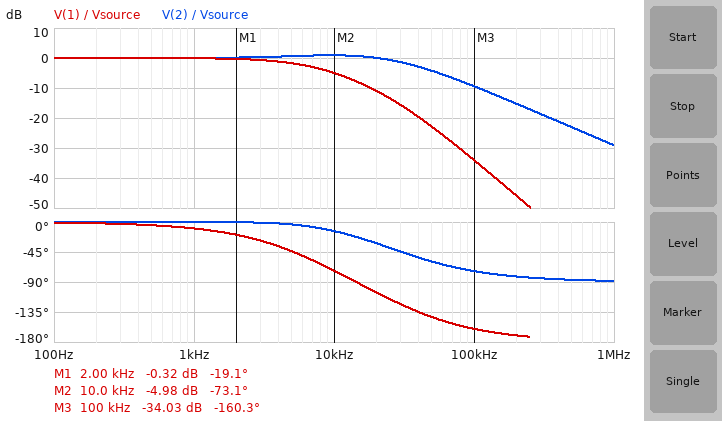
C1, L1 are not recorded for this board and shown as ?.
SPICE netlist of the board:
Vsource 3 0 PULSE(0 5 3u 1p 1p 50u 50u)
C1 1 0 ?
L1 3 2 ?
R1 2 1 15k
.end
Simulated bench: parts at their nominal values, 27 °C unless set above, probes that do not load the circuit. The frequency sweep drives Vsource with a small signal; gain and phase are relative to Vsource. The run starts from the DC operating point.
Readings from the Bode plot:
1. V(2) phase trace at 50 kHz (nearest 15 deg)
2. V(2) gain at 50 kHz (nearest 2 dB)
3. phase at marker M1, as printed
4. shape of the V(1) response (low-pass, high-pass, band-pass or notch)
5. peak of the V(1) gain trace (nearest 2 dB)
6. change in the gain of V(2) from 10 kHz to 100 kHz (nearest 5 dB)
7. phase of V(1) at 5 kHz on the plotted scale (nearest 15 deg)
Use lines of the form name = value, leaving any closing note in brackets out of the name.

V(2) phase trace at 50 kHz = -60 deg
V(2) gain at 50 kHz = -4 dB
phase at marker M1, as printed = -19.1 deg
shape of the V(1) response = low-pass
peak of the V(1) gain trace = 0 dB
change in the gain of V(2) from 10 kHz to 100 kHz = -10 dB
phase of V(1) at 5 kHz on the plotted scale = -45 deg
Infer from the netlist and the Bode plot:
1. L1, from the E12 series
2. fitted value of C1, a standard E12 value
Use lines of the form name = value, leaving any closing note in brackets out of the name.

L1, from the E12 series = 68 mH
fitted value of C1, a standard E12 value = 1.8 nF
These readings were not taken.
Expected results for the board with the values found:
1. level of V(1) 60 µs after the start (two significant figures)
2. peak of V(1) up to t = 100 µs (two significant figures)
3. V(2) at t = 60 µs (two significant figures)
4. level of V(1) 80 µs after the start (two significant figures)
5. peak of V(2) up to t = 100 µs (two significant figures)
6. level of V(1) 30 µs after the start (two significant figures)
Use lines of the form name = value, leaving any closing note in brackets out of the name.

level of V(1) 60 µs after the start = 4.5 V
peak of V(1) up to t = 100 µs = 4.9 V
V(2) at t = 60 µs = 5.1 V
level of V(1) 80 µs after the start = 4.8 V
peak of V(2) up to t = 100 µs = 5.5 V
level of V(1) 30 µs after the start = 3.1 V
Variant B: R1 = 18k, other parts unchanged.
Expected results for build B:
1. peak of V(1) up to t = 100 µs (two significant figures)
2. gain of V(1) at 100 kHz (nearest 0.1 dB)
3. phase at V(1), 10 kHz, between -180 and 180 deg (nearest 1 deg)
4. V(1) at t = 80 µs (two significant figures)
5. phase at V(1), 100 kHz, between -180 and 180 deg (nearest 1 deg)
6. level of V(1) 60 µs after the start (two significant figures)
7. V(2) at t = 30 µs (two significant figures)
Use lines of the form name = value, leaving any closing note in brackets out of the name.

peak of V(1) up to t = 100 µs = 4.8 V
gain of V(1) at 100 kHz = -34.2 dB
phase at V(1), 10 kHz, between -180 and 180 deg = -76 deg
V(1) at t = 80 µs = 4.6 V
phase at V(1), 100 kHz, between -180 and 180 deg = -157 deg
level of V(1) 60 µs after the start = 4.2 V
V(2) at t = 30 µs = 5.3 V
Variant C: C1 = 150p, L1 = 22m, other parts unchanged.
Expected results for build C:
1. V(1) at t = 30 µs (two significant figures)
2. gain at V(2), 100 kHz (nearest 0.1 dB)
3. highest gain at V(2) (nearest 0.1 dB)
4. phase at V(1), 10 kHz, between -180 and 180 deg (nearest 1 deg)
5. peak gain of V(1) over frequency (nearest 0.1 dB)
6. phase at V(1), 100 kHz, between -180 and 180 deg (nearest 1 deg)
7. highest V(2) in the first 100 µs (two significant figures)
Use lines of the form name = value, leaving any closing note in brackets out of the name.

V(1) at t = 30 µs = 5.0 V
gain at V(2), 100 kHz = 1.6 dB
highest gain at V(2) = 2.5 dB
phase at V(1), 10 kHz, between -180 and 180 deg = -8 deg
peak gain of V(1) over frequency = 0.2 dB
phase at V(1), 100 kHz, between -180 and 180 deg = -102 deg
highest V(2) in the first 100 µs = 6.2 V
